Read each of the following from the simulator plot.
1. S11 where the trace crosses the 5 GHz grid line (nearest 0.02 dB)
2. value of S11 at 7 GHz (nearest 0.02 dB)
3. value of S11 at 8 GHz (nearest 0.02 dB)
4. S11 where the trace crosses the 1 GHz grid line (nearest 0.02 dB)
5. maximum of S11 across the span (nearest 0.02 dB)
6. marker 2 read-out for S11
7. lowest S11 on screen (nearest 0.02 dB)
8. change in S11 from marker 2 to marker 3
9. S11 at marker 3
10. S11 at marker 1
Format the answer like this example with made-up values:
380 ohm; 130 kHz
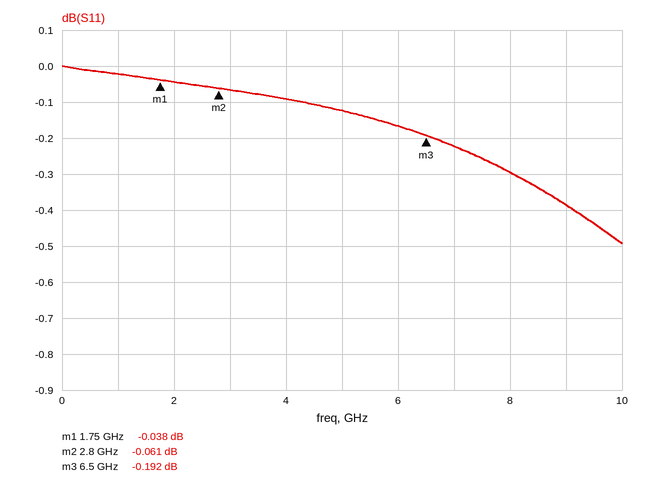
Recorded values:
-0.12 dB; -0.22 dB; -0.30 dB; -0.02 dB; 0.00 dB; -0.061 dB; -0.50 dB; -0.131 dB; -0.192 dB; -0.038 dB
